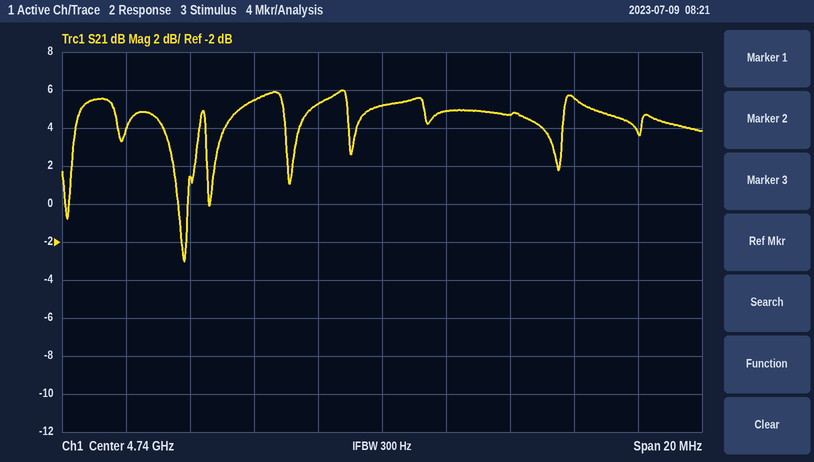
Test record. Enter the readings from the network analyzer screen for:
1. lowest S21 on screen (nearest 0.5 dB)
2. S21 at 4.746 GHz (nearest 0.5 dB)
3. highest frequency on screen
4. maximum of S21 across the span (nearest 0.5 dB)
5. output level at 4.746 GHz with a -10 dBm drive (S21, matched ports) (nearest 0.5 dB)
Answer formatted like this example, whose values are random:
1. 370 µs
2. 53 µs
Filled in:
1. -3.0 dB
2. 5.5 dB
3. 4.75 GHz
4. 6.0 dB
5. -4.5 dBm
